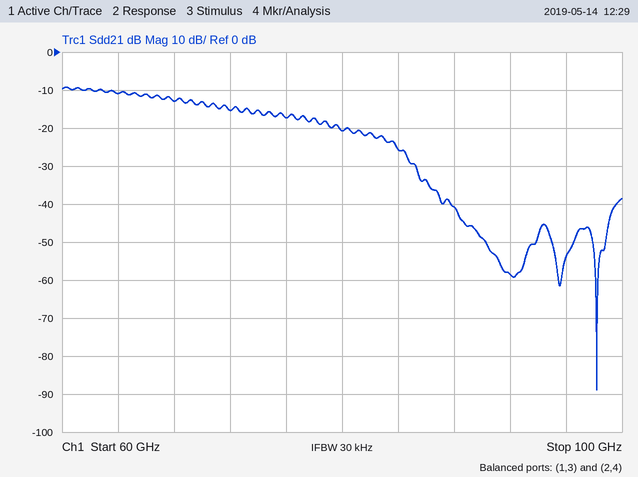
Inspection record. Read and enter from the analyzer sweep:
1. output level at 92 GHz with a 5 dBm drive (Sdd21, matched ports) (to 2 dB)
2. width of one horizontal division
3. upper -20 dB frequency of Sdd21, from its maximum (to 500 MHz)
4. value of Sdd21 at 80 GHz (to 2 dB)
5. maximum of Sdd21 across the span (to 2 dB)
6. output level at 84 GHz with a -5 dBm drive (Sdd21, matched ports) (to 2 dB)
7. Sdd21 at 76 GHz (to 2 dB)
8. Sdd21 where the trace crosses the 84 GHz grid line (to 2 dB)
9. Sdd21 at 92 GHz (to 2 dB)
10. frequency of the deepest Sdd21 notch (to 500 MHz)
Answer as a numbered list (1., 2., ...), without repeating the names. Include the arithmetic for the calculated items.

1. 5 dBm + (-58 dB) = -54 dBm
2. 4 GHz
3. 85.0 GHz
4. -20 dB
5. -10 dB
6. -5 dBm + (-26 dB) = -30 dBm
7. -18 dB
8. -26 dB
9. -58 dB
10. 98.0 GHz
